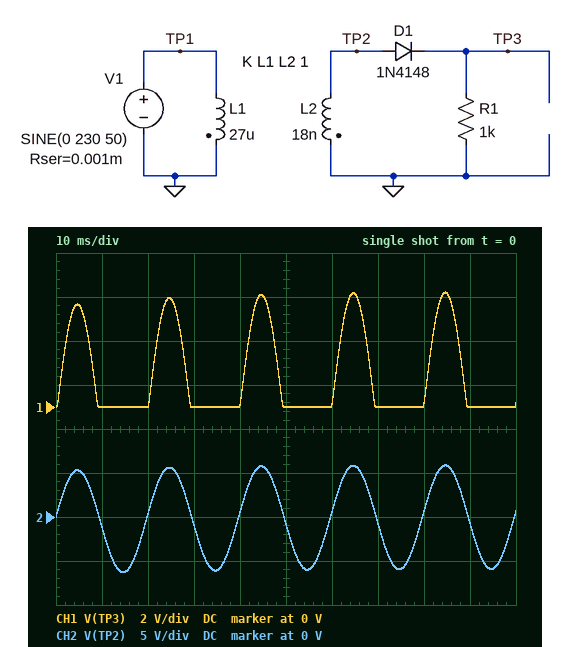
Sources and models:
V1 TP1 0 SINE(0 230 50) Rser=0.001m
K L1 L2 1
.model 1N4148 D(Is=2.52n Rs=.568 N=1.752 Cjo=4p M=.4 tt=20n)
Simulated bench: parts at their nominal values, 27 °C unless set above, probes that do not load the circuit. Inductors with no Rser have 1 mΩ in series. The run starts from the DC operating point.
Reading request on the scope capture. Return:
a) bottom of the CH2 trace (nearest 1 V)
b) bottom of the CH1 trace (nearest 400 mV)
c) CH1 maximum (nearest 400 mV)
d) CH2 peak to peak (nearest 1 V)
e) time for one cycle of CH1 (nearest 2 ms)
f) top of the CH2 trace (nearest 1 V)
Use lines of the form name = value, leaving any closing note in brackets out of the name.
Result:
bottom of the CH2 trace = -6 V
bottom of the CH1 trace = 0 V
CH1 maximum = 5.2 V
CH2 peak to peak = 12 V
time for one cycle of CH1 = 20 ms
top of the CH2 trace = 6 V
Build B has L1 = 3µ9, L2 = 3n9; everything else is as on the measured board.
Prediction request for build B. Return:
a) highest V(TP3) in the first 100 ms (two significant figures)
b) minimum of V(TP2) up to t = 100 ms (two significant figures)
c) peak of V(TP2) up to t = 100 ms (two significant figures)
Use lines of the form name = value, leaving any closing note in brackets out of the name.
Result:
highest V(TP3) in the first 100 ms = 5.0 V
minimum of V(TP2) up to t = 100 ms = -5.8 V
peak of V(TP2) up to t = 100 ms = 5.6 V
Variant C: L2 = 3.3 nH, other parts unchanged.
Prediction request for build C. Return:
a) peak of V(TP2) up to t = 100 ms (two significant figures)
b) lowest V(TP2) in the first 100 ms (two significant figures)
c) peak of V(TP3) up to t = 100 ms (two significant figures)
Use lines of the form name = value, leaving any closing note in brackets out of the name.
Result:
peak of V(TP2) up to t = 100 ms = 2.5 V
lowest V(TP2) in the first 100 ms = -2.7 V
peak of V(TP3) up to t = 100 ms = 1.9 V
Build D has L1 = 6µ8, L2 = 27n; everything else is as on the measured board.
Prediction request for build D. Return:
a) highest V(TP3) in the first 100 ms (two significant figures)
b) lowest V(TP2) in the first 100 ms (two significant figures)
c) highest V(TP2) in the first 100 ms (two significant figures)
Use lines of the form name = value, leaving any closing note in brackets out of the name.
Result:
highest V(TP3) in the first 100 ms = 12 V
lowest V(TP2) in the first 100 ms = -14 V
highest V(TP2) in the first 100 ms = 13 V
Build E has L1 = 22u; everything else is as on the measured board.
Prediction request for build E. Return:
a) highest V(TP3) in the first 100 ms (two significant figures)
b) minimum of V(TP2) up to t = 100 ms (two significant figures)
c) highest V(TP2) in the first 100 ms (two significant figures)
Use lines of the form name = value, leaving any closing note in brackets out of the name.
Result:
highest V(TP3) in the first 100 ms = 5.8 V
minimum of V(TP2) up to t = 100 ms = -7.0 V
highest V(TP2) in the first 100 ms = 6.5 V
